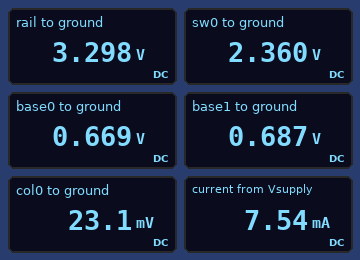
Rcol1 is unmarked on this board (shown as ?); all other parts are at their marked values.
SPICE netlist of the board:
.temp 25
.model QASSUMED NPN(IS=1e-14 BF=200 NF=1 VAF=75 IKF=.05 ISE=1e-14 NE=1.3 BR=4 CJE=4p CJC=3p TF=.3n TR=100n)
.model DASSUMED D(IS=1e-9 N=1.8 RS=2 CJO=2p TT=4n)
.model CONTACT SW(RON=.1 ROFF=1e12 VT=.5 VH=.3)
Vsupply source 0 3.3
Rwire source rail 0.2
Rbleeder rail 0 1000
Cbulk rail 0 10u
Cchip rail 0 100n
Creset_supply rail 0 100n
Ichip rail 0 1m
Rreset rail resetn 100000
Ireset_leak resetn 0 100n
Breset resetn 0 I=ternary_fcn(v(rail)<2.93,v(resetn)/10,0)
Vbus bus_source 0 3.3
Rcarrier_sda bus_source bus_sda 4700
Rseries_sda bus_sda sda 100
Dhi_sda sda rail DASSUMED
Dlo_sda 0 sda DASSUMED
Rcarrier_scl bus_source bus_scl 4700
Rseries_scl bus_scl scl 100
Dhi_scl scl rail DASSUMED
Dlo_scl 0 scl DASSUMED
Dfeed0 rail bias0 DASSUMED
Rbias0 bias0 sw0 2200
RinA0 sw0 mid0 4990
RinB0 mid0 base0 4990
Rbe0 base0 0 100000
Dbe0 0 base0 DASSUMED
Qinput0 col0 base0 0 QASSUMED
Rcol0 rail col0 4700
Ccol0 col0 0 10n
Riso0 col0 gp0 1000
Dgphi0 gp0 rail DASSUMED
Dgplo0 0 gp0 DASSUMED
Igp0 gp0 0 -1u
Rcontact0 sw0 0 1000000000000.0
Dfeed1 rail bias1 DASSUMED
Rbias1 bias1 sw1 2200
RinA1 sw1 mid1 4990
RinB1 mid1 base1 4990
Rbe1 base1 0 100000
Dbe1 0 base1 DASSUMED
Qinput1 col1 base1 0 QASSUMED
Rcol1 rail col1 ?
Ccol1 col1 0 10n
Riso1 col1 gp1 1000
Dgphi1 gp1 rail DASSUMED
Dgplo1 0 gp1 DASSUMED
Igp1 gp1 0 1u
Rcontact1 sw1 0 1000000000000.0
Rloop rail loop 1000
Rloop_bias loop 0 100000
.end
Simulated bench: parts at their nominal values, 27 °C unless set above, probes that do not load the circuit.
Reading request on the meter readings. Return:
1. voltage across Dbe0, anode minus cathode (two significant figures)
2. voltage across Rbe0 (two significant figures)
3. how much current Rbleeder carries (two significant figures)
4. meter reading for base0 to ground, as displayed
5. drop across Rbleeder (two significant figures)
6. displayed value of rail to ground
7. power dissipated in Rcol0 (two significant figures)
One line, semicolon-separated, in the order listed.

-670 mV; 670 mV; 3.3 mA; 0.669 V; 3.3 V; 3.298 V; 2.3 mW
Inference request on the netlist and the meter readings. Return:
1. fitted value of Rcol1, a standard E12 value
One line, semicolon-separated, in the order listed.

1.5 kΩ
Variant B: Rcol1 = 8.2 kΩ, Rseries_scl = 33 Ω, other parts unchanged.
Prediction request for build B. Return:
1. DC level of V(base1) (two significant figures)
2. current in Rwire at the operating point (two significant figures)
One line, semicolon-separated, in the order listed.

660 mV; 5.8 mA
